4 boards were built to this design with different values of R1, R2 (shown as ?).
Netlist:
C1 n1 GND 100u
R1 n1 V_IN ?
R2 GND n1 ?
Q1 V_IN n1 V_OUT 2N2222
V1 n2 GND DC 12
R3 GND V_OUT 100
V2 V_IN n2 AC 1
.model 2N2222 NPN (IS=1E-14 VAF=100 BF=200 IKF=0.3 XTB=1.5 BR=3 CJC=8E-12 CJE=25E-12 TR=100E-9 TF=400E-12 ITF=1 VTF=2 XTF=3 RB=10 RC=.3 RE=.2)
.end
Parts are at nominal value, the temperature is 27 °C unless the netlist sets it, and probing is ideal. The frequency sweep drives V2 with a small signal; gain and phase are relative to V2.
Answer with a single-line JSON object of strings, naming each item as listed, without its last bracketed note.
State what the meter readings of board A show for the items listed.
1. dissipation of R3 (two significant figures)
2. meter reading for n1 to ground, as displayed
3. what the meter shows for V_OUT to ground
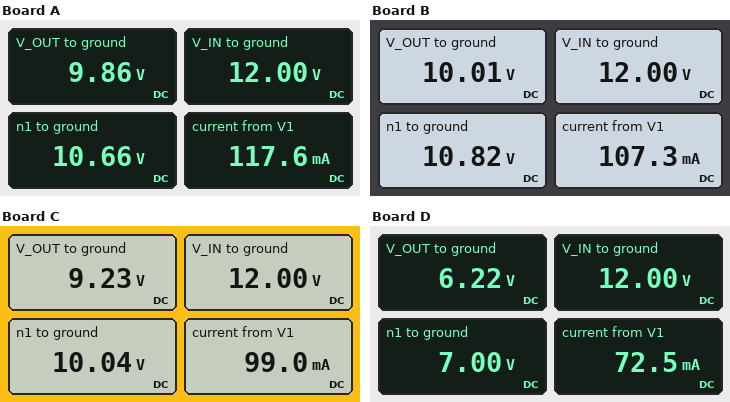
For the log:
{"dissipation of R3": "970 mW", "meter reading for n1 to ground, as displayed": "10.66 V", "what the meter shows for V_OUT to ground": "9.86 V"}
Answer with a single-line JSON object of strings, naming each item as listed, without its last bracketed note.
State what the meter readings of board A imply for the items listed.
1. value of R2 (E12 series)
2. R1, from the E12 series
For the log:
{"value of R2": "560 Ω", "R1, from the E12 series": "68 Ω"}
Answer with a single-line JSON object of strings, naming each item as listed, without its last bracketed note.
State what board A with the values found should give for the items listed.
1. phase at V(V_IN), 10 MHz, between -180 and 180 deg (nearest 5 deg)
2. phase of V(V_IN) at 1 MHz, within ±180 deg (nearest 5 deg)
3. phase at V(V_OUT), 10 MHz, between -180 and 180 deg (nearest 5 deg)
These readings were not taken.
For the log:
{"phase at V(V_IN), 10 MHz, between -180 and 180 deg": "0 deg", "phase of V(V_IN) at 1 MHz, within ±180 deg": "0 deg", "phase at V(V_OUT), 10 MHz, between -180 and 180 deg": "85 deg"}
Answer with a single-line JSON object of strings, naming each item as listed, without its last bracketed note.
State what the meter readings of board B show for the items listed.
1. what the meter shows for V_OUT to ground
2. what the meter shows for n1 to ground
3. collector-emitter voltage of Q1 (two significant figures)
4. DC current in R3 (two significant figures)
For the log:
{"what the meter shows for V_OUT to ground": "10.01 V", "what the meter shows for n1 to ground": "10.82 V", "collector-emitter voltage of Q1": "2.0 V", "DC current in R3": "100 mA"}
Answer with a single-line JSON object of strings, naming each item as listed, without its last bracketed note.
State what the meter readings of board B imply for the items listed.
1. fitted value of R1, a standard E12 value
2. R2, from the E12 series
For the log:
{"fitted value of R1, a standard E12 value": "150 Ω", "R2, from the E12 series": "1.5 kΩ"}
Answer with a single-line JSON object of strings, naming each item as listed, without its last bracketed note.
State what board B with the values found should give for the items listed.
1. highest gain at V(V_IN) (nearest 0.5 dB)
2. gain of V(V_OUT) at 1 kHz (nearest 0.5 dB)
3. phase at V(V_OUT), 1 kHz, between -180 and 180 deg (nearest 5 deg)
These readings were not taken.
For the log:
{"highest gain at V(V_IN)": "0 dB", "gain of V(V_OUT) at 1 kHz": "-39.5 dB", "phase at V(V_OUT), 1 kHz, between -180 and 180 deg": "-85 deg"}
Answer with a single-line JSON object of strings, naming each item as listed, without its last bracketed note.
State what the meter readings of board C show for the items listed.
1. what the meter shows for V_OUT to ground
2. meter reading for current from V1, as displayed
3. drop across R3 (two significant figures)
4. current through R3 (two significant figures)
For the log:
{"what the meter shows for V_OUT to ground": "9.23 V", "meter reading for current from V1, as displayed": "99.0 mA", "drop across R3": "9.2 V", "current through R3": "92 mA"}
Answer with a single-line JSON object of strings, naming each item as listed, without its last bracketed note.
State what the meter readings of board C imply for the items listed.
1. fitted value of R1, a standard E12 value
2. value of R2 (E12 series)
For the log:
{"fitted value of R1, a standard E12 value": "270 Ω", "value of R2": "1.5 kΩ"}
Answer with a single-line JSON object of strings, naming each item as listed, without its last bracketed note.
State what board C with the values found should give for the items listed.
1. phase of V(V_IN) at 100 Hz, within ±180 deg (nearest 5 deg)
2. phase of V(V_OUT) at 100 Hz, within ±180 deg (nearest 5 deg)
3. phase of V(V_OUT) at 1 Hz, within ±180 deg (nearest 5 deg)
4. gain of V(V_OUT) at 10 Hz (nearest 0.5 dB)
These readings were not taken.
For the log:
{"phase of V(V_IN) at 100 Hz, within ±180 deg": "0 deg", "phase of V(V_OUT) at 100 Hz, within ±180 deg": "-85 deg", "phase of V(V_OUT) at 1 Hz, within ±180 deg": "-10 deg", "gain of V(V_OUT) at 10 Hz": "-6.5 dB"}
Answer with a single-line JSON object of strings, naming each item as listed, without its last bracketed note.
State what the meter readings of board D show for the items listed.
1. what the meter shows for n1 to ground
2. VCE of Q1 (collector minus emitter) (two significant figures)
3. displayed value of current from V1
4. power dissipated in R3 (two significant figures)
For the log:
{"what the meter shows for n1 to ground": "7.00 V", "VCE of Q1 (collector minus emitter)": "5.8 V", "displayed value of current from V1": "72.5 mA", "power dissipated in R3": "390 mW"}
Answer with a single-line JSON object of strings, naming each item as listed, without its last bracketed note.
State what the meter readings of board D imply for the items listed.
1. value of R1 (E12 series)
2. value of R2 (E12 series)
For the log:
{"value of R1": "470 Ω", "value of R2": "680 Ω"}
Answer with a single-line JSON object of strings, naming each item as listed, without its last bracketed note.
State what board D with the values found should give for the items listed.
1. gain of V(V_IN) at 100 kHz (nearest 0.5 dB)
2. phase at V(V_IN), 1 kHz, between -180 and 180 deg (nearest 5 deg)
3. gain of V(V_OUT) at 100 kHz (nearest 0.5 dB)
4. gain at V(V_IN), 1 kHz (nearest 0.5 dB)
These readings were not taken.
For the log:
{"gain of V(V_IN) at 100 kHz": "0 dB", "phase at V(V_IN), 1 kHz, between -180 and 180 deg": "0 deg", "gain of V(V_OUT) at 100 kHz": "-70.0 dB", "gain at V(V_IN), 1 kHz": "0 dB"}
